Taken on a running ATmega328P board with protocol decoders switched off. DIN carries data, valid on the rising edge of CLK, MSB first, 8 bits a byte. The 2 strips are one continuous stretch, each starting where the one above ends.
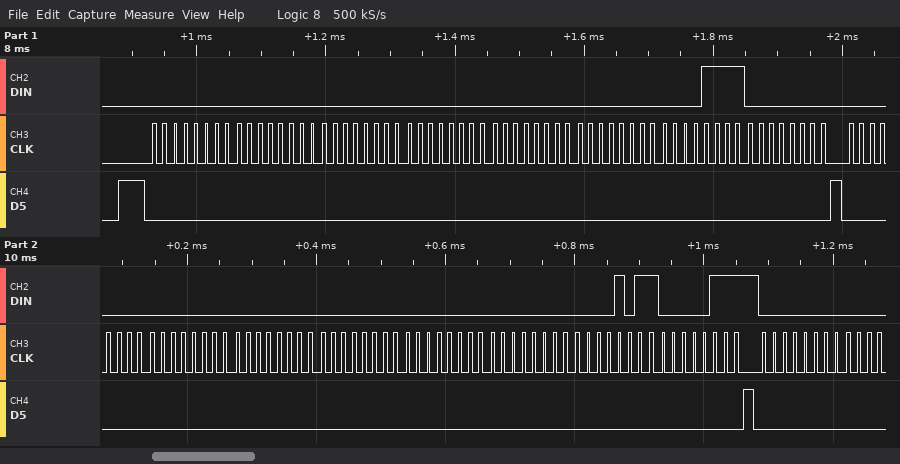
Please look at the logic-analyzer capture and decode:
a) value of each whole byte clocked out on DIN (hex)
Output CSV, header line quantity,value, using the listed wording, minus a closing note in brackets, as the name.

quantity,value
value of each whole byte clocked out on DIN,00 00 00 00 00 00 0F 00 00 00 00 00 00 00 0B 07 00
